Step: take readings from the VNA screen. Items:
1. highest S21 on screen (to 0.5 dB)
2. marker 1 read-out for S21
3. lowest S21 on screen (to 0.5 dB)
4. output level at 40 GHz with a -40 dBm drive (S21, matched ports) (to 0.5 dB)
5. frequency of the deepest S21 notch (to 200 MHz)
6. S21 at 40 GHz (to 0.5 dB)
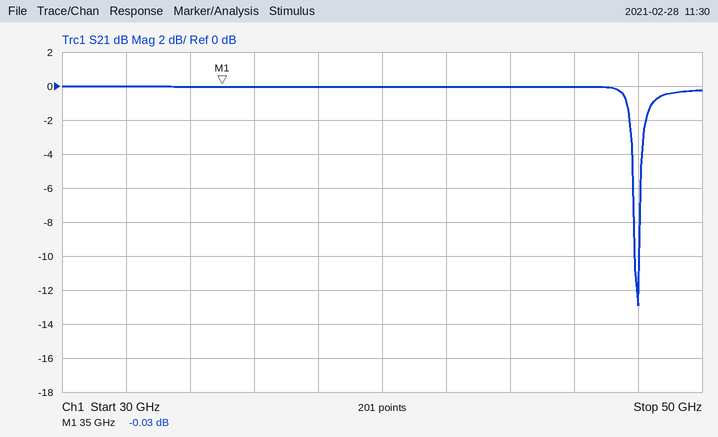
0.0 dB
-0.03 dB
-13.0 dB
-40.0 dBm
48.0 GHz
0.0 dB
